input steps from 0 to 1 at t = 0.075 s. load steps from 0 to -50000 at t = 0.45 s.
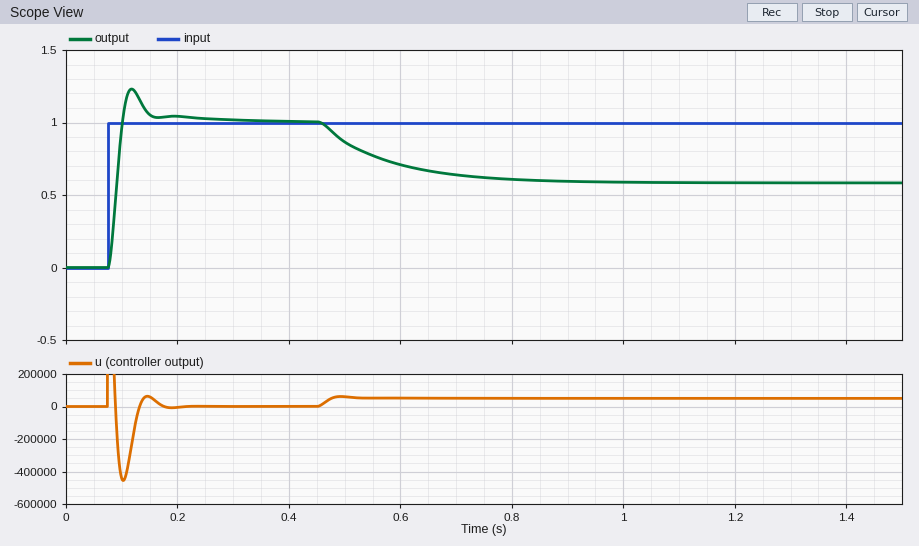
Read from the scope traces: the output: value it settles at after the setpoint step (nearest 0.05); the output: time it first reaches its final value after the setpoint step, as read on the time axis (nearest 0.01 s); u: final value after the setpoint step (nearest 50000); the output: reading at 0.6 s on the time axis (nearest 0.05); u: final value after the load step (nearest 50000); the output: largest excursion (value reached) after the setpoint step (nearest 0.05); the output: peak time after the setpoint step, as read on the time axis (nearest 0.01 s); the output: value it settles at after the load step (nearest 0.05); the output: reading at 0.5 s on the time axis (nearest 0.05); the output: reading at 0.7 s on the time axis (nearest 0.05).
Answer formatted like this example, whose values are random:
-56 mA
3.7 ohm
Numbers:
1.00
0.10 s
0
0.70
50000
1.25
0.12 s
0.60
0.85
0.65
